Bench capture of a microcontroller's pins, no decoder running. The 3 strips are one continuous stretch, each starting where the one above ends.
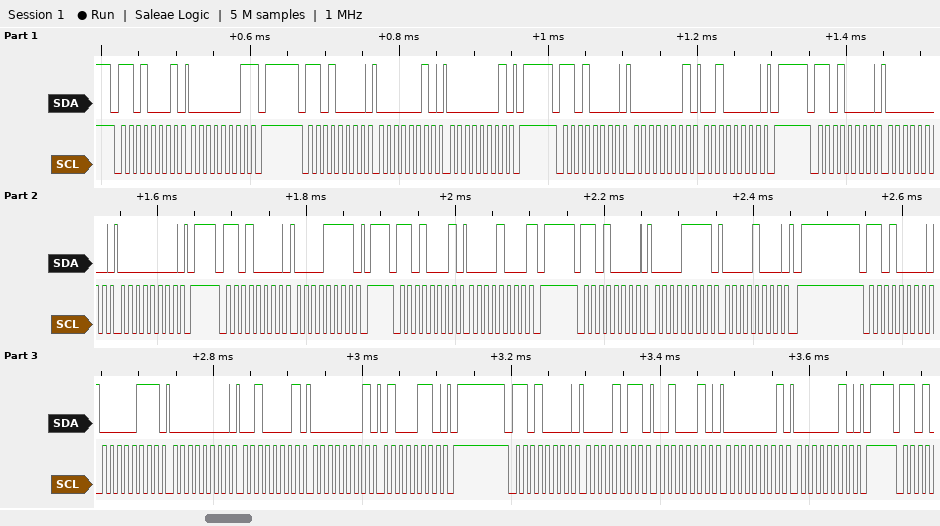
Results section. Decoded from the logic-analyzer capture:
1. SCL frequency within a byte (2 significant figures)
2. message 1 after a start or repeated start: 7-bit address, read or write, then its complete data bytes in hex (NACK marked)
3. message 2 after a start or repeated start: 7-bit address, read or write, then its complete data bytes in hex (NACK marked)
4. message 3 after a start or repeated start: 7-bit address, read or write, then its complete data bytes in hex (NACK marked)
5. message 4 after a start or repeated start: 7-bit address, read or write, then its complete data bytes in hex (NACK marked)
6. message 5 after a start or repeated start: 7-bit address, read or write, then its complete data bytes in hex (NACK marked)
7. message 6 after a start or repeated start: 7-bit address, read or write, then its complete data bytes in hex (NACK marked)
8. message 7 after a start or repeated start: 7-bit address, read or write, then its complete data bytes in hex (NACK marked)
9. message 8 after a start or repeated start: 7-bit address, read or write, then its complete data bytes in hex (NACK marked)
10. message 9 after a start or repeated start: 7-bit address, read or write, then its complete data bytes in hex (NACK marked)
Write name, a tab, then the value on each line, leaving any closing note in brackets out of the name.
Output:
SCL frequency within a byte	100 kHz
message 1 after a start or repeated start: 7-bit address, read or write, then its complete data bytes in hex	0x68 read: 01 NACK
message 2 after a start or repeated start: 7-bit address, read or write, then its complete data bytes in hex	0x68 write: 02 01
message 3 after a start or repeated start: 7-bit address, read or write, then its complete data bytes in hex	0x68 write: 01 20
message 4 after a start or repeated start: 7-bit address, read or write, then its complete data bytes in hex	0x68 write: 00 00
message 5 after a start or repeated start: 7-bit address, read or write, then its complete data bytes in hex	0x68 write: 0F
message 6 after a start or repeated start: 7-bit address, read or write, then its complete data bytes in hex	0x68 read: 08 NACK
message 7 after a start or repeated start: 7-bit address, read or write, then its complete data bytes in hex	0x68 write: 0F 08
message 8 after a start or repeated start: 7-bit address, read or write, then its complete data bytes in hex	0x68 write: 07 00 21 01 46
message 9 after a start or repeated start: 7-bit address, read or write, then its complete data bytes in hex	0x68 write: 0B 22 01 02
